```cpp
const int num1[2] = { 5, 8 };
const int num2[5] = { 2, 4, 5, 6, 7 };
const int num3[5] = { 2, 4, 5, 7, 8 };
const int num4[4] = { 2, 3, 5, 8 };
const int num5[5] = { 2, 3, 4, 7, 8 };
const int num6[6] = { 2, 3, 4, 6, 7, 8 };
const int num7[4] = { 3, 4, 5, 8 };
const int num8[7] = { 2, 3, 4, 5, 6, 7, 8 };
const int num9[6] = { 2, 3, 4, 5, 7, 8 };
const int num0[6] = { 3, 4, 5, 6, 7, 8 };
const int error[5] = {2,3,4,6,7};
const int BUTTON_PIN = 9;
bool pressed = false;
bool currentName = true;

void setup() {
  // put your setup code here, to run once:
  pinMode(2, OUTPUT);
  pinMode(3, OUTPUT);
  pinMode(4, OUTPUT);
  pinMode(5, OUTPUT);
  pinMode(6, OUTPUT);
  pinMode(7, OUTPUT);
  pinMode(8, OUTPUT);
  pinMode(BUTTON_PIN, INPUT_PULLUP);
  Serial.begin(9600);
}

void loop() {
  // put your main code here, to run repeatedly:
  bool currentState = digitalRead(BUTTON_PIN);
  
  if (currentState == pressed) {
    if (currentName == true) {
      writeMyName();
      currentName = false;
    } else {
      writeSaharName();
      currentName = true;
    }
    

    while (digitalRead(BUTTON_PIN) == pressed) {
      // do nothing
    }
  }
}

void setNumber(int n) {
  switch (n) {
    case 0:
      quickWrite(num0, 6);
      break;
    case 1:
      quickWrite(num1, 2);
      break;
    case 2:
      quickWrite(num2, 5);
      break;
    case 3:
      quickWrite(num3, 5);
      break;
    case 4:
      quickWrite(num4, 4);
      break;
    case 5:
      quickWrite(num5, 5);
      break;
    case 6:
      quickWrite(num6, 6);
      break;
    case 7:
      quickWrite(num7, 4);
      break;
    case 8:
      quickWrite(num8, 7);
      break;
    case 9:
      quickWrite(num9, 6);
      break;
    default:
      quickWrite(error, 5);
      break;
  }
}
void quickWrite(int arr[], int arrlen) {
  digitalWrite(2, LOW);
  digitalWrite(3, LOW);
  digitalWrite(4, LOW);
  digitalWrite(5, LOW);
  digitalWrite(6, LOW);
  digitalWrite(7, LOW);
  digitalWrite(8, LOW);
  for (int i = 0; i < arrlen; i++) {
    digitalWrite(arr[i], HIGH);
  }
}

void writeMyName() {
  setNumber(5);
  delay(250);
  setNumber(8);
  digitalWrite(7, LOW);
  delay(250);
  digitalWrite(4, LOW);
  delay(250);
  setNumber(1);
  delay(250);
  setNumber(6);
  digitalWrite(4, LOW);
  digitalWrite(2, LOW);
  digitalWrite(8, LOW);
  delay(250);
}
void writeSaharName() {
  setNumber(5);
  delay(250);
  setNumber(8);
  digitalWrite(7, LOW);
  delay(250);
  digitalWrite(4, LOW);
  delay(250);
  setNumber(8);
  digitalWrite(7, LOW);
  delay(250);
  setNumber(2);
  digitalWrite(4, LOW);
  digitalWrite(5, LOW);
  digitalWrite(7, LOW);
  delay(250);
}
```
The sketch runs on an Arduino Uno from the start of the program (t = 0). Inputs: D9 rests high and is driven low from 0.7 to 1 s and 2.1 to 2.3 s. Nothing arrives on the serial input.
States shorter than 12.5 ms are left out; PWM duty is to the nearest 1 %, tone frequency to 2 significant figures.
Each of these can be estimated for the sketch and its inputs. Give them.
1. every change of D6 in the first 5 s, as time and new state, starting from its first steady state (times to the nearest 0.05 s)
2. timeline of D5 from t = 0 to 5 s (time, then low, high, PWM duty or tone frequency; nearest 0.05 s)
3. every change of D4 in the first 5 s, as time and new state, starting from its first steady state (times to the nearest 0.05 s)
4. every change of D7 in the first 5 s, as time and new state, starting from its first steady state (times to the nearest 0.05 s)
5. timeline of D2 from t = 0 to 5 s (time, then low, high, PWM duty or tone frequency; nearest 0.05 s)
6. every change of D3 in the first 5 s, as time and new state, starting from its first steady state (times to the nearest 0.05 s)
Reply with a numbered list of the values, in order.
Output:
1. 0 s low; 0.95 s high; 1.45 s low; 1.7 s high; 2.1 s low; 2.35 s high
2. 0 s low; 0.95 s high; 1.7 s low; 2.35 s high; 3.1 s low
3. 0 s low; 0.7 s high; 1.2 s low; 2.1 s high; 2.6 s low; 2.85 s high; 3.1 s low
4. 0 s low; 0.7 s high; 0.95 s low; 1.7 s high; 2.35 s low
5. 0 s low; 0.7 s high; 1.45 s low; 2.1 s high
6. 0 s low; 0.7 s high; 1.45 s low; 1.7 s high; 3.1 s low
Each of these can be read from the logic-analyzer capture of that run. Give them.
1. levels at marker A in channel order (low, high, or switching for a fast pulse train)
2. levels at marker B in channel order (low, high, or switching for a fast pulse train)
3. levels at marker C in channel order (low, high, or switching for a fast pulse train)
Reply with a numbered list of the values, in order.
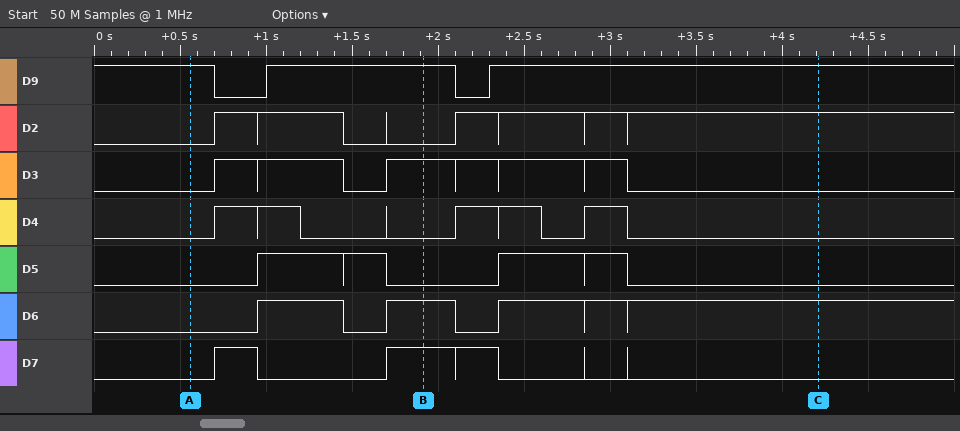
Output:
1. D9 high, D2 low, D3 low, D4 low, D5 low, D6 low, D7 low
2. D9 high, D2 low, D3 high, D4 low, D5 low, D6 high, D7 high
3. D9 high, D2 high, D3 low, D4 low, D5 low, D6 high, D7 low
